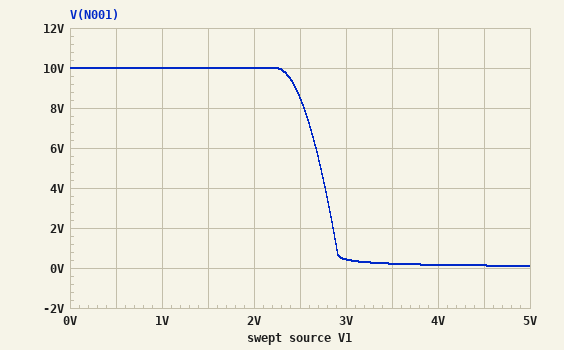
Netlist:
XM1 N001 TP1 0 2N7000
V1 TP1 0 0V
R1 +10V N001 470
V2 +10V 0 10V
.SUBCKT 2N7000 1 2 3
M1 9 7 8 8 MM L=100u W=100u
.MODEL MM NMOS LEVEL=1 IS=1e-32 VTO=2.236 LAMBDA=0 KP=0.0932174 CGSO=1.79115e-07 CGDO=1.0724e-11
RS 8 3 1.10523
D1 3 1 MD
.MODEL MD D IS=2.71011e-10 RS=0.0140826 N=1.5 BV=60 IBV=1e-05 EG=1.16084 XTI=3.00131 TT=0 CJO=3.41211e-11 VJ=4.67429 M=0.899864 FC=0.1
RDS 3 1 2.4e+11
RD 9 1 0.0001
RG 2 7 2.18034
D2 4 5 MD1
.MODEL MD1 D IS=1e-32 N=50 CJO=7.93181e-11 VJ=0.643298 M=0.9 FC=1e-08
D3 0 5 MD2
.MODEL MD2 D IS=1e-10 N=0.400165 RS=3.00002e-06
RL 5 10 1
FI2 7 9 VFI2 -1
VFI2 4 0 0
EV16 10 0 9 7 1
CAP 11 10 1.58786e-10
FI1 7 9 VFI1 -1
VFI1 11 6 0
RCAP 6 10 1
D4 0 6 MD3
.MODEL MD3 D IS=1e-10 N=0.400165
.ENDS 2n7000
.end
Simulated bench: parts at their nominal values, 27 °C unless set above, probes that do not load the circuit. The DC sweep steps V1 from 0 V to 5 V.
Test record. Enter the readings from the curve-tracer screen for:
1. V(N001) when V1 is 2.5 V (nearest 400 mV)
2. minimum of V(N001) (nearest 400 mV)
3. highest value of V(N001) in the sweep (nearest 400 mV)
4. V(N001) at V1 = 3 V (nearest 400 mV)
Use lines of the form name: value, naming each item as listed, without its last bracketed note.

V(N001) when V1 is 2.5 V: 8.4 V
minimum of V(N001): 0 V
highest value of V(N001) in the sweep: 10.0 V
V(N001) at V1 = 3 V: 400 mV
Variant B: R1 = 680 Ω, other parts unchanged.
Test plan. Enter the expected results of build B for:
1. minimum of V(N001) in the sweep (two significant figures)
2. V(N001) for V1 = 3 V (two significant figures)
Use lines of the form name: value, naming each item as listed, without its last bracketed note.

minimum of V(N001) in the sweep: 74 mV
V(N001) for V1 = 3 V: 260 mV
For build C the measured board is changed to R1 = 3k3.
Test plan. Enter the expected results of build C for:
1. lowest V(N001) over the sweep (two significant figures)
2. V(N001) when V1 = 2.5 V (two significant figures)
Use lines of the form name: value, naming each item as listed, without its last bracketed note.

lowest V(N001) over the sweep: 15 mV
V(N001) when V1 = 2.5 V: 200 mV
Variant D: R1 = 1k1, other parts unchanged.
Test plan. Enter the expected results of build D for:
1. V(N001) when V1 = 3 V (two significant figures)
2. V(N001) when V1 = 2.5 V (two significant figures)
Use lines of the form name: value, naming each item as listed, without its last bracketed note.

V(N001) when V1 = 3 V: 150 mV
V(N001) when V1 = 2.5 V: 6.5 V
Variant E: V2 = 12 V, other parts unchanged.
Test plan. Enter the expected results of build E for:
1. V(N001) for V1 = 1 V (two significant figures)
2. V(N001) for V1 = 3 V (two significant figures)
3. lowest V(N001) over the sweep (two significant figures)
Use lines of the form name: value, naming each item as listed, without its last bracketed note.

V(N001) for V1 = 1 V: 12 V
V(N001) for V1 = 3 V: 610 mV
lowest V(N001) over the sweep: 130 mV
